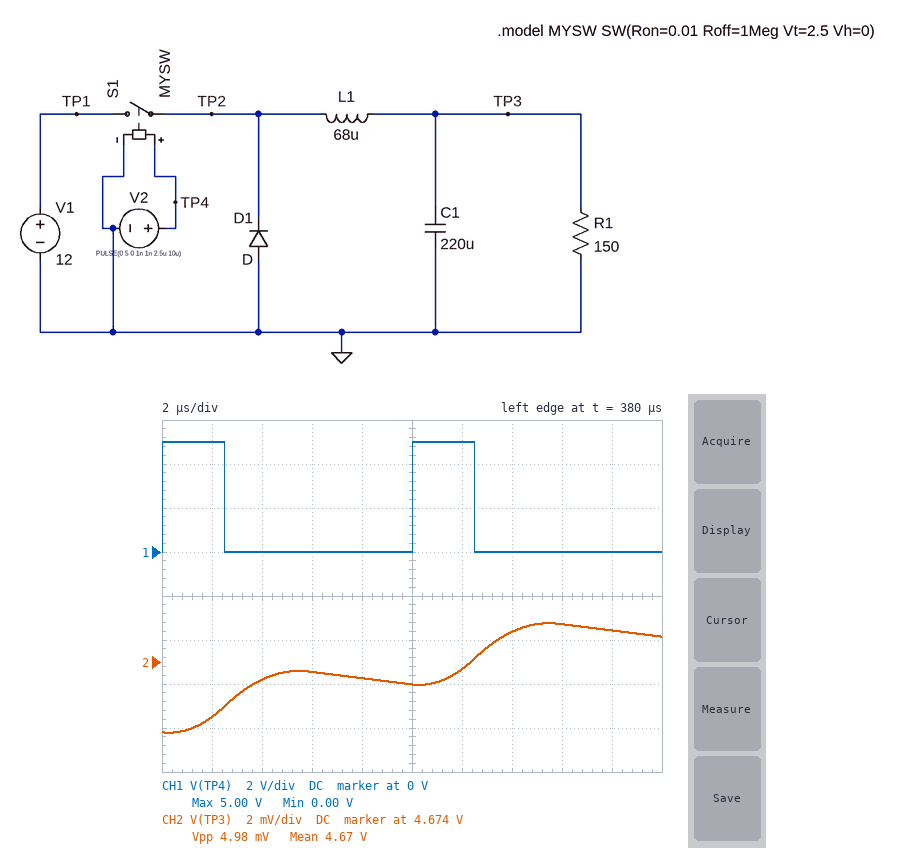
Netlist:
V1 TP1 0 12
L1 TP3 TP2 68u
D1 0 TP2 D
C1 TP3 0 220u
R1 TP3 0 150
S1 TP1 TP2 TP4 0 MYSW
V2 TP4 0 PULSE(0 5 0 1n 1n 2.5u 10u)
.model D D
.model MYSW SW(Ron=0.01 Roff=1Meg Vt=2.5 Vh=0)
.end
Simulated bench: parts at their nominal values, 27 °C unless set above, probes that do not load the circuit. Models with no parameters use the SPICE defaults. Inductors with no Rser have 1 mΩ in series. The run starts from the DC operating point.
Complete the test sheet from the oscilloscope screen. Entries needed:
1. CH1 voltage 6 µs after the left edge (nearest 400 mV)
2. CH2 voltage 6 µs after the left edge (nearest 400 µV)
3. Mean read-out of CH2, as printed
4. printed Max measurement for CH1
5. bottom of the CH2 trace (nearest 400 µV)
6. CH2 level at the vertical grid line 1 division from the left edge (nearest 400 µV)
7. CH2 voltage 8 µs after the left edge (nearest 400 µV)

0 V
4.6736 V
4.67 V
5.00 V
4.6708 V
4.6716 V
4.6732 V
